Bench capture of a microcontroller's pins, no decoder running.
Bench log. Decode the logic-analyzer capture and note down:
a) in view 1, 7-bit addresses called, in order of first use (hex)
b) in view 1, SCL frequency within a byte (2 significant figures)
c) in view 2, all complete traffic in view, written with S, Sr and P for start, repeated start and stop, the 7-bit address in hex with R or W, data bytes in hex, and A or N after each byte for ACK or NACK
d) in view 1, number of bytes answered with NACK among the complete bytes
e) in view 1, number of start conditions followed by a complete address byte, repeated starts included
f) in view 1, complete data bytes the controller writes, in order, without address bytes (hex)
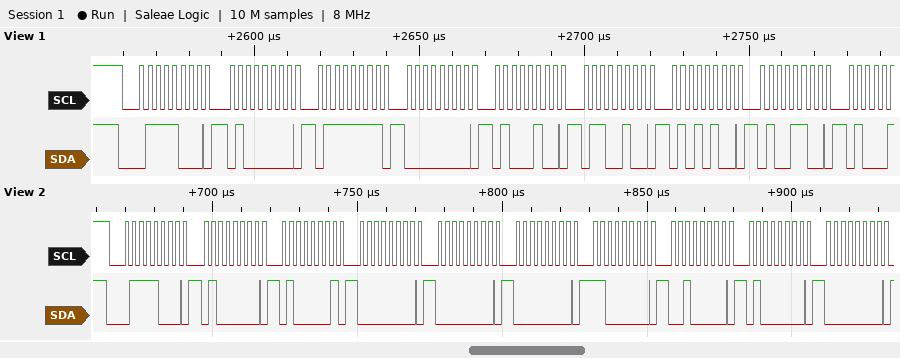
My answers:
0x3C
400 kHz
S 3CW A 40 A 41 A 00 A 00 A 00 A C0 A 20 A 40 A 00 A
0
1
40 7F 00 44 64 54 4C
